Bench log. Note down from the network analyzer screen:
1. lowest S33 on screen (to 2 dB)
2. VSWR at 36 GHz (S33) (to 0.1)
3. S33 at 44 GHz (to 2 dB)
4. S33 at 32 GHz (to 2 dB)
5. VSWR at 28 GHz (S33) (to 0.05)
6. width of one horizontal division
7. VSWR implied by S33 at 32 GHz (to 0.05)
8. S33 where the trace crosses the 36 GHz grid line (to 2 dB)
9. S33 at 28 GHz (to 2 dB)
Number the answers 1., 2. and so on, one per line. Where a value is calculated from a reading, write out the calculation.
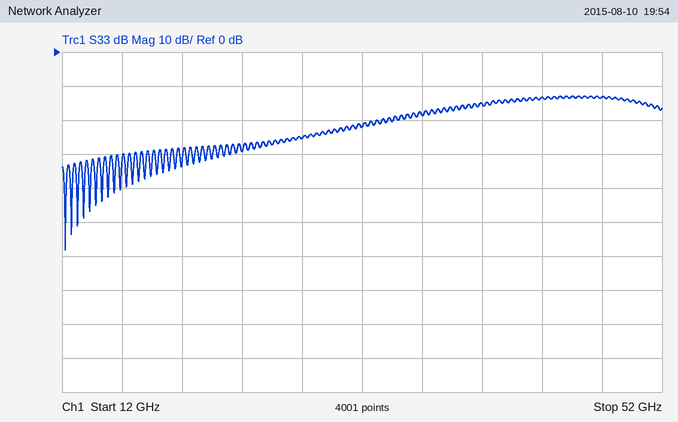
1. -58 dB
2. |Γ| = 10^(-18/20) = 0.1259; VSWR = (1 + 0.1259)/(1 − 0.1259) ≈ 1.3
3. -14 dB
4. -22 dB
5. |Γ| = 10^(-26/20) = 0.0501; VSWR = (1 + 0.0501)/(1 − 0.0501) ≈ 1.11, so 1.10 to the nearest 0.05
6. 4 GHz
7. |Γ| = 10^(-22/20) = 0.0794; VSWR = (1 + 0.0794)/(1 − 0.0794) ≈ 1.17, so 1.15 to the nearest 0.05
8. -18 dB
9. -26 dB
